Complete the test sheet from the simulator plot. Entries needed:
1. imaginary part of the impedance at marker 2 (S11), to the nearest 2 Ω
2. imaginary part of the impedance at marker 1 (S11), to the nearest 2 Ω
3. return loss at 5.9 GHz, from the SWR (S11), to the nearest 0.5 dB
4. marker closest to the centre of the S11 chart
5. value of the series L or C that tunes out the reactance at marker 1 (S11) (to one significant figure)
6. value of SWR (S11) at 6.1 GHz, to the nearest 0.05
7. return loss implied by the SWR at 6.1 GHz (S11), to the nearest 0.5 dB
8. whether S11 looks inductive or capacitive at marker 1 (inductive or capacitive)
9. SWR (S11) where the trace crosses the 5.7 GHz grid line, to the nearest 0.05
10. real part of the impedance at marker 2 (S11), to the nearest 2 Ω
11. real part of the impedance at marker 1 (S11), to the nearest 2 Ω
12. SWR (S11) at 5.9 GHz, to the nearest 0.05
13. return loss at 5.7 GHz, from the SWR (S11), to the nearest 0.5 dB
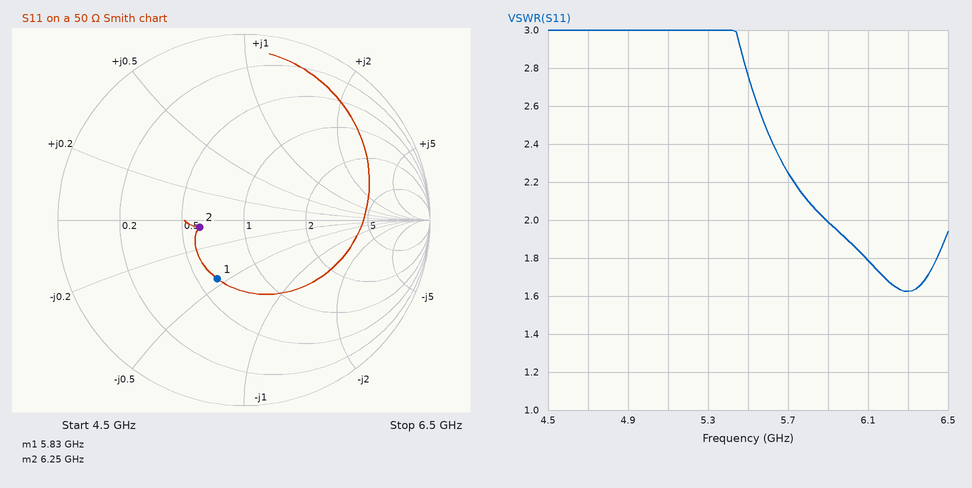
-2 Ω
-22 Ω
9.5 dB
marker 2
600 pH
1.80
11.0 dB
capacitive
2.25
30 Ω
32 Ω
2.00
8.5 dB
